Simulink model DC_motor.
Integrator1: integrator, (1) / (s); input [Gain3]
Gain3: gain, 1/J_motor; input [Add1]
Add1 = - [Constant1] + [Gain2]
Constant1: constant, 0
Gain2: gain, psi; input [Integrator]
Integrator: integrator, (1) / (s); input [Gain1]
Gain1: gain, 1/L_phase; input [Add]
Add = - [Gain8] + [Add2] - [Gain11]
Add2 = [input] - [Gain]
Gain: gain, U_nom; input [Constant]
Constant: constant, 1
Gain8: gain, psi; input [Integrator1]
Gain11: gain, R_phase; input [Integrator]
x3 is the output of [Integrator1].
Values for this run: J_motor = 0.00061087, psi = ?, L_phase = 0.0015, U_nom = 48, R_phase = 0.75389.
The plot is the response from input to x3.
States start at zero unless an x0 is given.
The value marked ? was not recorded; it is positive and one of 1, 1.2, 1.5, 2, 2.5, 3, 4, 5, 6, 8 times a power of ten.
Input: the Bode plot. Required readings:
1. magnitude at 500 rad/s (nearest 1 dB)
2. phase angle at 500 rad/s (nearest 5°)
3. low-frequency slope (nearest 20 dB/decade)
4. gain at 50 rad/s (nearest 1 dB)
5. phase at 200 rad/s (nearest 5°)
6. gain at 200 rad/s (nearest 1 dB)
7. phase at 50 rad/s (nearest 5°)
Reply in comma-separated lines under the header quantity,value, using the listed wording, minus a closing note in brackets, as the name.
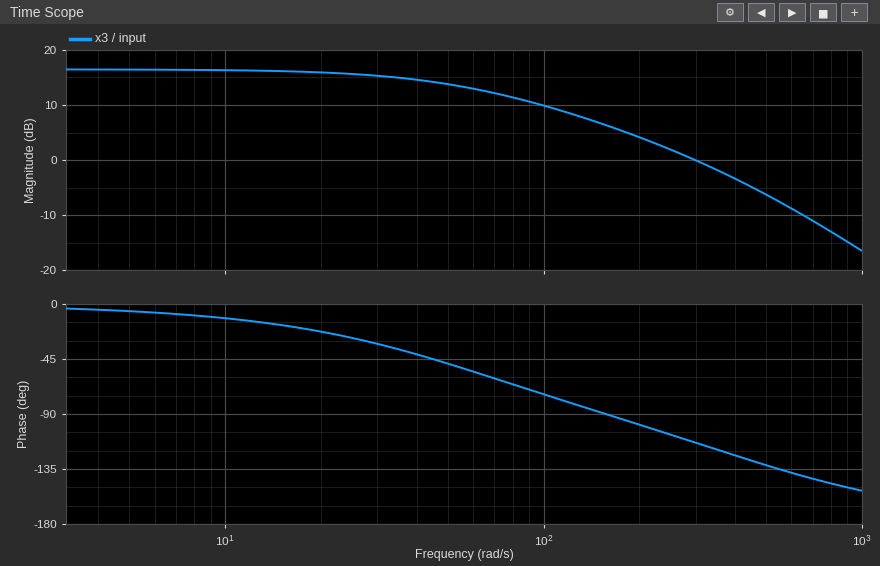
quantity,value
magnitude at 500 rad/s,-6 dB
phase angle at 500 rad/s,-130°
low-frequency slope,0 dB/decade
gain at 50 rad/s,14 dB
phase at 200 rad/s,-100°
gain at 200 rad/s,4 dB
phase at 50 rad/s,-50°
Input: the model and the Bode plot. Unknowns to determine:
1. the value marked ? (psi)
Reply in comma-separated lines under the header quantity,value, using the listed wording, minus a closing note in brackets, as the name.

quantity,value
the value marked ?,0.15
